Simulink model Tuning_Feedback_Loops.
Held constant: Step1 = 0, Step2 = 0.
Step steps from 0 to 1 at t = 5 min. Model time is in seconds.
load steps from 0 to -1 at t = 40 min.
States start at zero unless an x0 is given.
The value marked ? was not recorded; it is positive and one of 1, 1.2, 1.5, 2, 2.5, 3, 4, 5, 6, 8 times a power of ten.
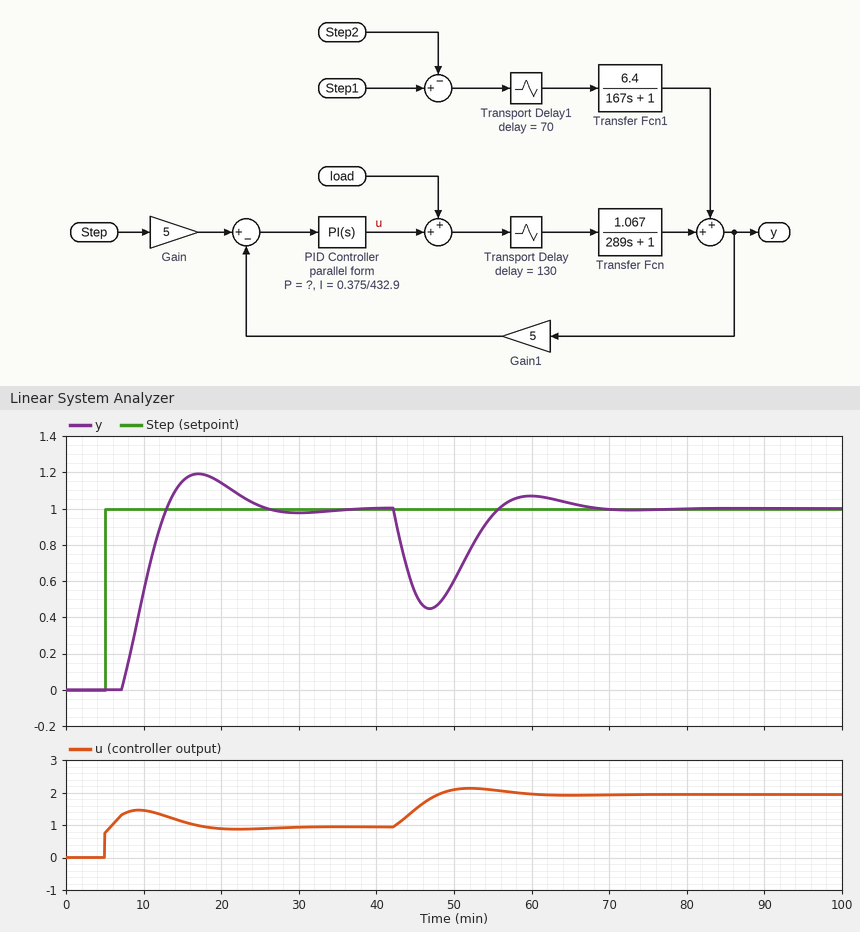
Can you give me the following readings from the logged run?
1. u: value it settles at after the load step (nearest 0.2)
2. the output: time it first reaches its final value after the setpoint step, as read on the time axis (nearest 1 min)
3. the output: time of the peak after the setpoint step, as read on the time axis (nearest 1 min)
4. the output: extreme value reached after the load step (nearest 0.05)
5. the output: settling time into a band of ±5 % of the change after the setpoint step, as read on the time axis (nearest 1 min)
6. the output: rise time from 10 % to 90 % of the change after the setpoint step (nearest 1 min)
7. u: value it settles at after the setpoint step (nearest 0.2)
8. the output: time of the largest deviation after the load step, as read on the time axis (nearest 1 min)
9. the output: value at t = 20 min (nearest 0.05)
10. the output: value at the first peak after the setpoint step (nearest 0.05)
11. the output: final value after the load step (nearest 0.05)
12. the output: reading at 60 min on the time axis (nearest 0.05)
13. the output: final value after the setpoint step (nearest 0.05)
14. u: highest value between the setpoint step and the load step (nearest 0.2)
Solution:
2.0
13 min
17 min
0.45
23 min
4 min
1.0
47 min
1.15
1.20
1.00
1.05
1.00
1.4
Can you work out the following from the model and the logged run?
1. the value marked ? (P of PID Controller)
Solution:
0.15
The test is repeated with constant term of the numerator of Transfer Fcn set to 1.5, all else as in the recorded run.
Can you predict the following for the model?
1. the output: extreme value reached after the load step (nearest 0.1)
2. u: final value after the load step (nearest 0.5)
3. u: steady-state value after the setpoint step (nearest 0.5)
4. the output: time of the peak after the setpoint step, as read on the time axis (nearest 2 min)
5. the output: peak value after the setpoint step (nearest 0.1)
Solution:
0.3
1.5
0.5
14 min
1.3
